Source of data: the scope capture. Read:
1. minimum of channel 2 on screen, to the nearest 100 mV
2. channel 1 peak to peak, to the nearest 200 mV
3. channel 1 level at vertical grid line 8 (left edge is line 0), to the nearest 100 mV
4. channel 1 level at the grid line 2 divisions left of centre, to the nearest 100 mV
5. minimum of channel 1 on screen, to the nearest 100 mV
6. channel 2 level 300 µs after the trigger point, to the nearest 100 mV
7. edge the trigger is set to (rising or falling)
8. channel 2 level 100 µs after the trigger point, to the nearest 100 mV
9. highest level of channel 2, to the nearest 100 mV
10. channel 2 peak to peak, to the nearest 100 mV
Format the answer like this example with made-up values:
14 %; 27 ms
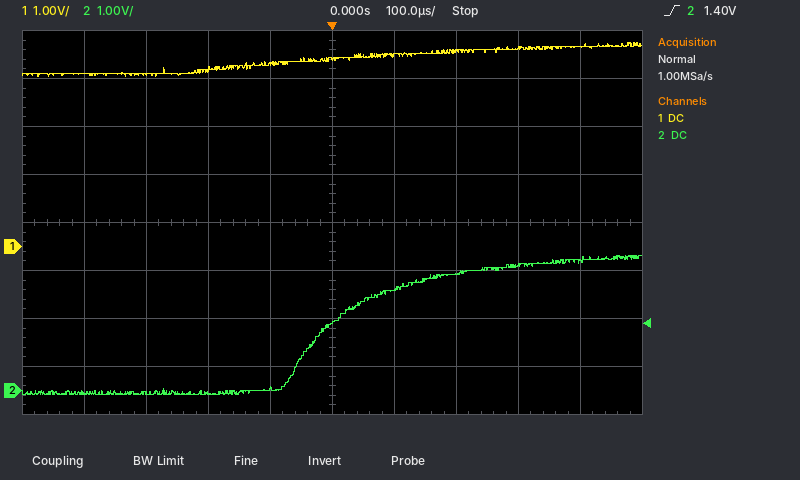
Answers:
-100 mV; 800 mV; 4.1 V; 3.7 V; 3.5 V; 2.6 V; rising; 2.1 V; 2.8 V; 2.9 V
